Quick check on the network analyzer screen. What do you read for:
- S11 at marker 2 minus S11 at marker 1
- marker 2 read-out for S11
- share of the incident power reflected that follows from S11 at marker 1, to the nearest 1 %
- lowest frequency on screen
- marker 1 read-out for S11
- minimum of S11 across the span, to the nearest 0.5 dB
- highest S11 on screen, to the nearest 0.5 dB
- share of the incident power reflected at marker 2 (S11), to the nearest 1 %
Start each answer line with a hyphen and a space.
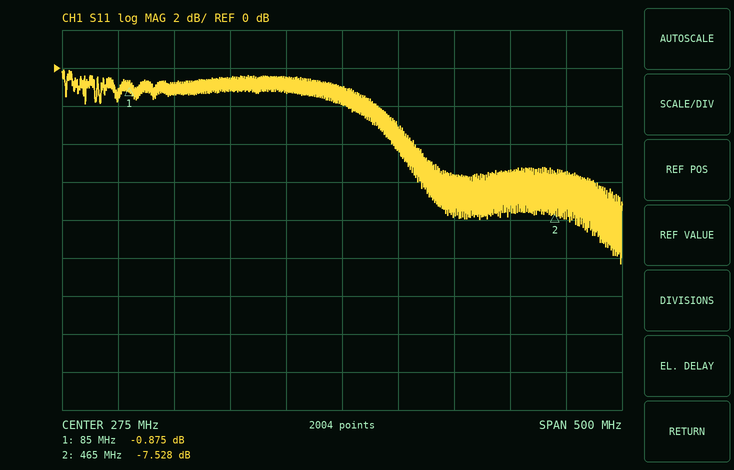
- -6.653 dB
- -7.528 dB
- 82 %
- 25 MHz
- -0.875 dB
- -10.5 dB
- 0.0 dB
- 18 %
